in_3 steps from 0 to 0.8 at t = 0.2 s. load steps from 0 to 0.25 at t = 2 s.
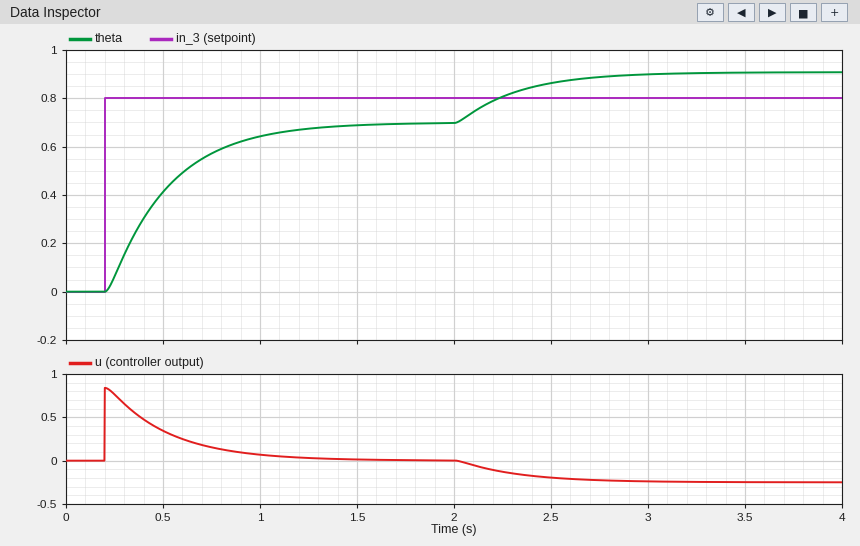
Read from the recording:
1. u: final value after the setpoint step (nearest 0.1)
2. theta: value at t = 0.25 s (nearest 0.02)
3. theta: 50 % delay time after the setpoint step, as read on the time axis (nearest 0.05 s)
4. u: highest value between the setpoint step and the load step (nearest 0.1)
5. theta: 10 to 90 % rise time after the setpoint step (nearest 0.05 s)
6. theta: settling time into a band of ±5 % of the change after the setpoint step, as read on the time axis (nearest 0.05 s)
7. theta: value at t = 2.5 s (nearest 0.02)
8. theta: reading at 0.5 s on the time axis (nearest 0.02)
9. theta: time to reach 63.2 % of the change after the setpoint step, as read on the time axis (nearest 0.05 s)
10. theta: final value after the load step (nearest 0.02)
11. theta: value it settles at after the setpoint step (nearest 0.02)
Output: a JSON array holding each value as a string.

["0.0", "0.06", "0.45 s", "0.8", "0.70 s", "1.15 s", "0.86", "0.42", "0.55 s", "0.90", "0.70"]
